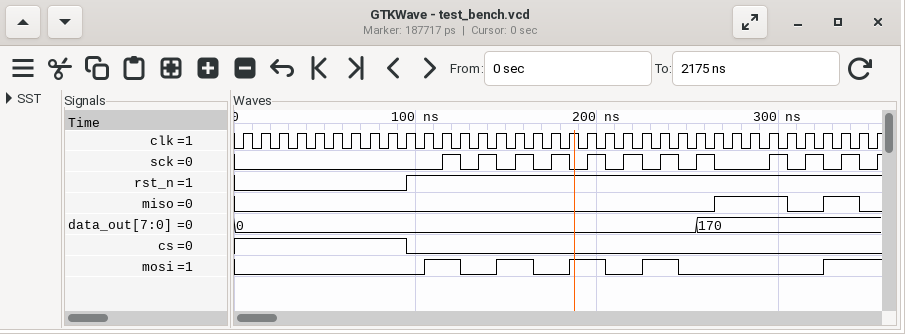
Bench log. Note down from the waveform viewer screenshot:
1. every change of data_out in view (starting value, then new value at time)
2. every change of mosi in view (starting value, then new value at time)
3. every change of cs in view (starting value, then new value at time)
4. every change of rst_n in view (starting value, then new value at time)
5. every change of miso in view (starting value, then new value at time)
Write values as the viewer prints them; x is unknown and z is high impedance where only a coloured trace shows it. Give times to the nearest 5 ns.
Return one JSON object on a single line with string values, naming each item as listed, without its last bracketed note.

{"every change of data_out in view": "0, 170 at 255 ns", "every change of mosi in view": "0, 1 at 105 ns, 0 at 125 ns, 1 at 145 ns, 0 at 165 ns, 1 at 185 ns, 0 at 205 ns, 1 at 225 ns, 0 at 245 ns, 1 at 325 ns", "every change of cs in view": "1, 0 at 95 ns", "every change of rst_n in view": "0, 1 at 95 ns", "every change of miso in view": "0, 1 at 265 ns, 0 at 305 ns, 1 at 325 ns, 0 at 345 ns"}
